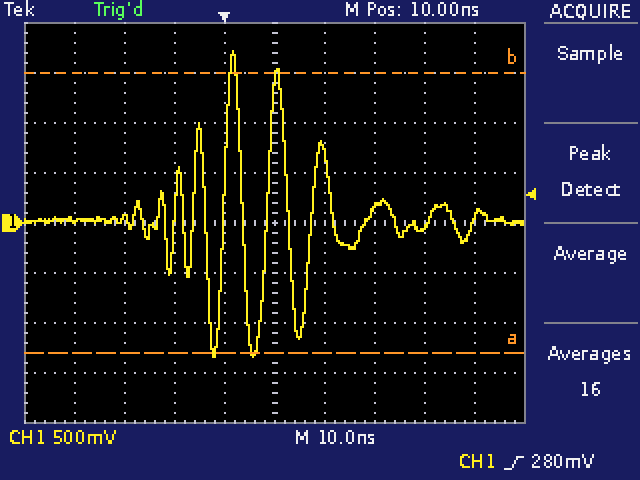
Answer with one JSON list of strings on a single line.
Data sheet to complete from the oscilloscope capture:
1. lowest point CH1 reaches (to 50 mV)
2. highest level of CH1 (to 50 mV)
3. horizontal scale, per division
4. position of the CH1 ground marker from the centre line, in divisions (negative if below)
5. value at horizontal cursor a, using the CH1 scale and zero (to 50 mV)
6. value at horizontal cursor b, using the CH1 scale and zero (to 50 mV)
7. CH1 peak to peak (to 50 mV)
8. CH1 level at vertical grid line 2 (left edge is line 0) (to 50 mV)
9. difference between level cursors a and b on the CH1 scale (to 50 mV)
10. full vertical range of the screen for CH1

["-1.35 V", "1.70 V", "10 ns", "0.0 div", "-1.30 V", "1.50 V", "3.05 V", "50 mV", "2.80 V", "4 V"]
